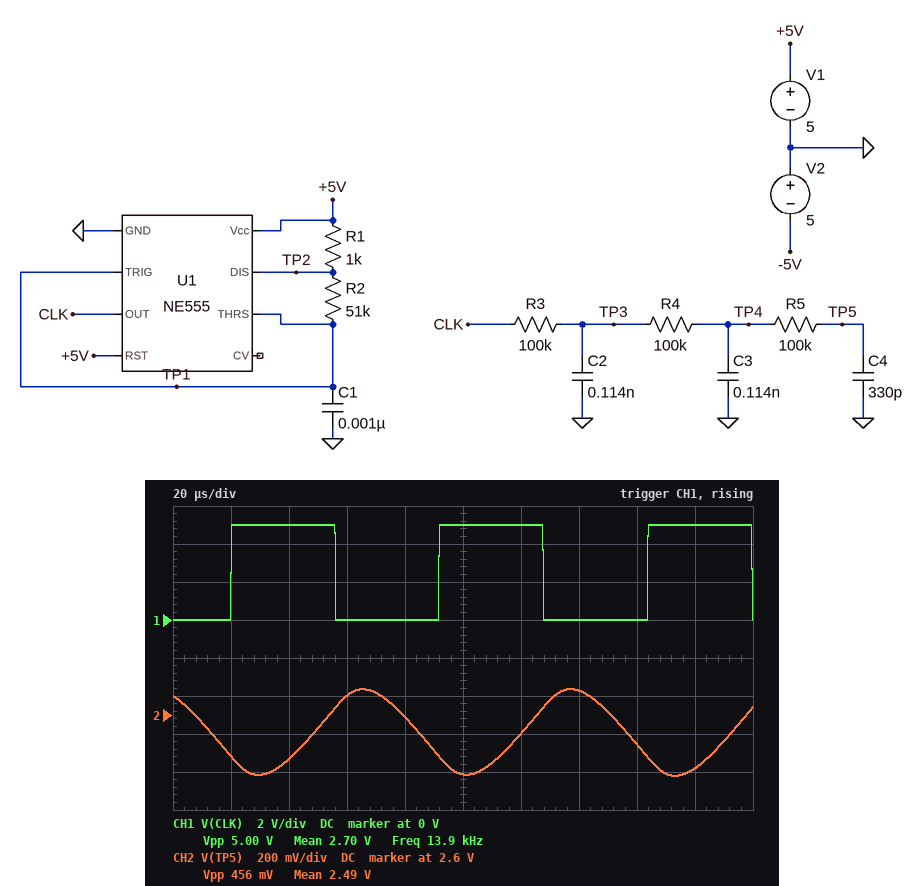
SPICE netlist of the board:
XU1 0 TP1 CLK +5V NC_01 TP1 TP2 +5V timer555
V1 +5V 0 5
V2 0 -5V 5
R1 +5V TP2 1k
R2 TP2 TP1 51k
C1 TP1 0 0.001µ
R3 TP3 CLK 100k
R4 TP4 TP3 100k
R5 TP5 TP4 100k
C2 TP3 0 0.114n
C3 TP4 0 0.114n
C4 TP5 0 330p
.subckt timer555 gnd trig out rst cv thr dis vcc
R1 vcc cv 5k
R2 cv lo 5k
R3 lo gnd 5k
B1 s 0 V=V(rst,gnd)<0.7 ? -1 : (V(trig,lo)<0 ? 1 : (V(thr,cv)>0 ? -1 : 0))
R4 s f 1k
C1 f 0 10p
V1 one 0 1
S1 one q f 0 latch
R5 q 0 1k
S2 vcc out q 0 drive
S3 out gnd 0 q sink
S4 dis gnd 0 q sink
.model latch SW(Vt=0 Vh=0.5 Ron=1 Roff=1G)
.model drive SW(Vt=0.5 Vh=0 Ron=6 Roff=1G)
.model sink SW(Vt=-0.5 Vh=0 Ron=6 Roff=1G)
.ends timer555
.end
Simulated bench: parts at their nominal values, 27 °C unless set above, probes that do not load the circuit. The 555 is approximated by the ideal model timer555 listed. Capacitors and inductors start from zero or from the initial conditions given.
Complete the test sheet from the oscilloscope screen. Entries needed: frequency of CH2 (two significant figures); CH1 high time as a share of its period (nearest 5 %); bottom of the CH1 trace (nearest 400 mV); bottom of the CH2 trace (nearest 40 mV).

14 kHz
50 %
0 V
2.28 V
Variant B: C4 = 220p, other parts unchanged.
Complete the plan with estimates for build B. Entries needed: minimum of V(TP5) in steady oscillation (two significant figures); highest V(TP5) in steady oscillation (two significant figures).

2.2 V
2.8 V
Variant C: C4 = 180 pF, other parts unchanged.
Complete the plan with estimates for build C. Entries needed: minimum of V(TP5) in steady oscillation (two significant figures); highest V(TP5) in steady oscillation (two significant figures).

2.1 V
2.9 V
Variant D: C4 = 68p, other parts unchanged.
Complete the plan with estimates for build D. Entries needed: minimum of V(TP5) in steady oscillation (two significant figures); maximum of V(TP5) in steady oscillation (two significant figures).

1.8 V
3.2 V
